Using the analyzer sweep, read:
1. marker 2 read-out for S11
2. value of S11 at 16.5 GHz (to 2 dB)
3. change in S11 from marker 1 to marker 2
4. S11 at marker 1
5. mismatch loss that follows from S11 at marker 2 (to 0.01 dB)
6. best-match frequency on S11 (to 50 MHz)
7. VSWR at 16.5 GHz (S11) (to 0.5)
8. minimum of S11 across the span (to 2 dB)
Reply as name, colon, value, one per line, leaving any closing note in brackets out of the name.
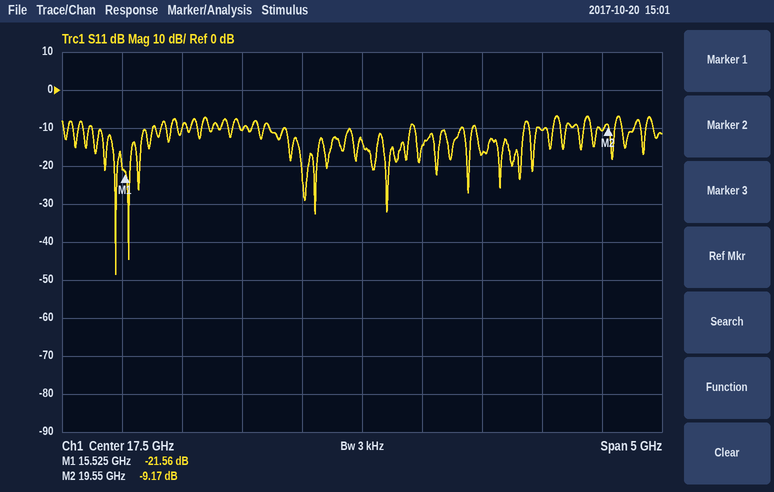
marker 2 read-out for S11: -9.17 dB
value of S11 at 16.5 GHz: -10 dB
change in S11 from marker 1 to marker 2: 12.39 dB
S11 at marker 1: -21.56 dB
mismatch loss that follows from S11 at marker 2: 0.56 dB
best-match frequency on S11: 15.45 GHz
VSWR at 16.5 GHz (S11): 2.0
minimum of S11 across the span: -48 dB
